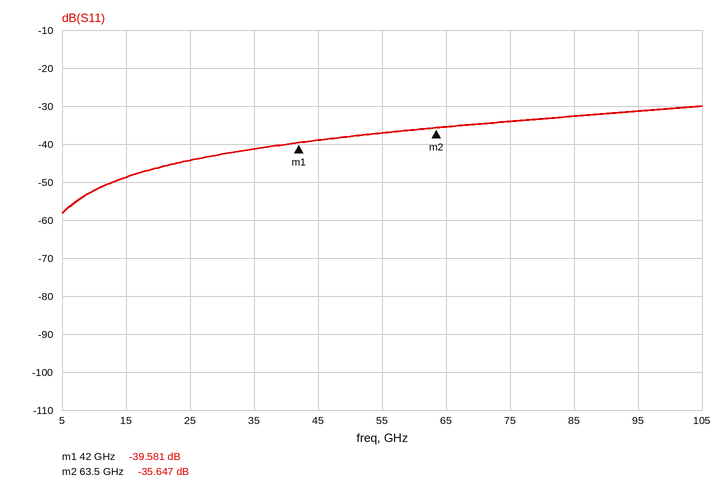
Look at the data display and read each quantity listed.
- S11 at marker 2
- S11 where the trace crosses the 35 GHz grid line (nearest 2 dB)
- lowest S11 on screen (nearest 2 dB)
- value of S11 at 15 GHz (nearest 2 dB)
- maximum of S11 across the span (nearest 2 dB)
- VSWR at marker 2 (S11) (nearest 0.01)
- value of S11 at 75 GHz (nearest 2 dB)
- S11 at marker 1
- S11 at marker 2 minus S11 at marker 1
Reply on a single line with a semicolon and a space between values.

-35.647 dB; -42 dB; -58 dB; -48 dB; -30 dB; 1.03; -34 dB; -39.581 dB; 3.934 dB
